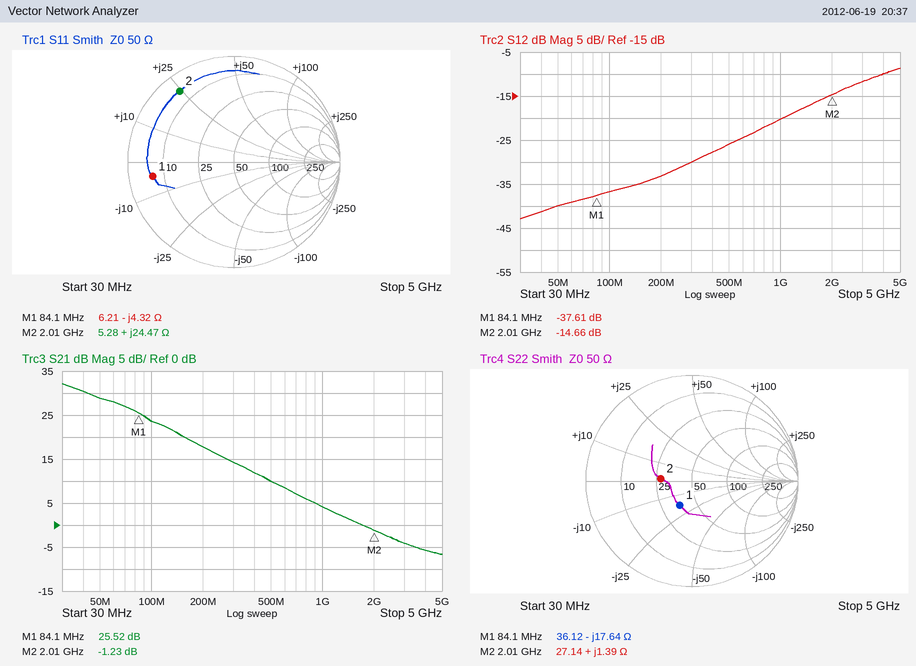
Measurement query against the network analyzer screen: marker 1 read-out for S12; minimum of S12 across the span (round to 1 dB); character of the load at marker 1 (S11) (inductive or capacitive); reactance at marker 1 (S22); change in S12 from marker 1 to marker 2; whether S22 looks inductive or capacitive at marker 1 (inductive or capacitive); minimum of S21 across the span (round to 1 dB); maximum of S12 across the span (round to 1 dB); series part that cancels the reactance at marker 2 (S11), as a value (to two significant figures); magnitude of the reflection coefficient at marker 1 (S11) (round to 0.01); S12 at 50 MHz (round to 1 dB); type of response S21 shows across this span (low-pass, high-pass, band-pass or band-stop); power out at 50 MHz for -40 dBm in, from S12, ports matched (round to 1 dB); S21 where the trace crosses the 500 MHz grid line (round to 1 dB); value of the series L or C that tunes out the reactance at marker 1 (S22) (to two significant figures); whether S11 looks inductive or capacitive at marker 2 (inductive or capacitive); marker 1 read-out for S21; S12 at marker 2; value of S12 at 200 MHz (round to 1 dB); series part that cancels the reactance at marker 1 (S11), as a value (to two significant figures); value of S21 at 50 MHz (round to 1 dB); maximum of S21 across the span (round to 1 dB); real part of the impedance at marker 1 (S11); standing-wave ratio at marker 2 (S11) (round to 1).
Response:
-37.61 dB
-43 dB
capacitive
-17.64 Ω
22.95 dB
capacitive
-7 dB
-9 dB
3.2 pF
0.78
-40 dB
low-pass
-80 dBm
10 dB
33 nH
inductive
25.52 dB
-14.66 dB
-33 dB
8.2 nH
29 dB
32 dB
6.21 Ω
12
